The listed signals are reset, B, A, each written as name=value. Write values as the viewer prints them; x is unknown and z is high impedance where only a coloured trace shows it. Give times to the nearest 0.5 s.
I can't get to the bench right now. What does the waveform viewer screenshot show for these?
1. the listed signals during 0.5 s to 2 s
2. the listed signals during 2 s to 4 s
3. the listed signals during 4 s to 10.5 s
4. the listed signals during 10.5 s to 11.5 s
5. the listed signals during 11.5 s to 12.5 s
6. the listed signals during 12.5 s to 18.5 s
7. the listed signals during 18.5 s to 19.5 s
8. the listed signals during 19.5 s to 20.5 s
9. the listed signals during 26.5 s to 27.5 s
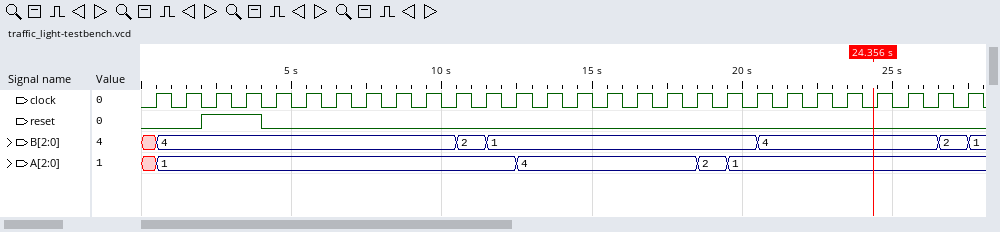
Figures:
reset=0, B=4, A=1
reset=1, B=4, A=1
reset=0, B=4, A=1
reset=0, B=2, A=1
reset=0, B=1, A=1
reset=0, B=1, A=4
reset=0, B=1, A=2
reset=0, B=1, A=1
reset=0, B=2, A=1
